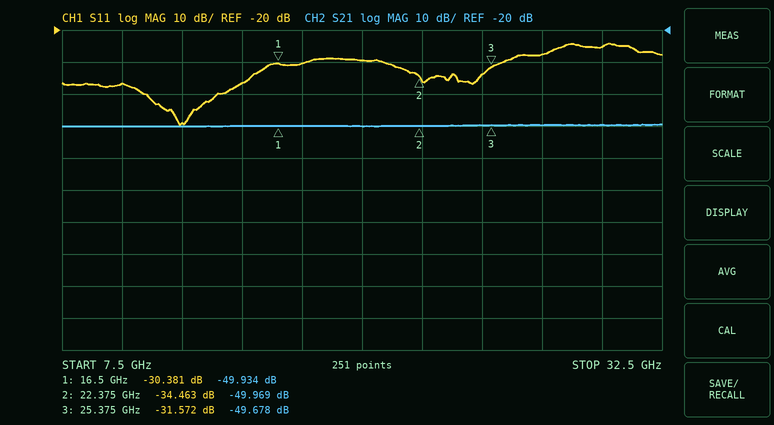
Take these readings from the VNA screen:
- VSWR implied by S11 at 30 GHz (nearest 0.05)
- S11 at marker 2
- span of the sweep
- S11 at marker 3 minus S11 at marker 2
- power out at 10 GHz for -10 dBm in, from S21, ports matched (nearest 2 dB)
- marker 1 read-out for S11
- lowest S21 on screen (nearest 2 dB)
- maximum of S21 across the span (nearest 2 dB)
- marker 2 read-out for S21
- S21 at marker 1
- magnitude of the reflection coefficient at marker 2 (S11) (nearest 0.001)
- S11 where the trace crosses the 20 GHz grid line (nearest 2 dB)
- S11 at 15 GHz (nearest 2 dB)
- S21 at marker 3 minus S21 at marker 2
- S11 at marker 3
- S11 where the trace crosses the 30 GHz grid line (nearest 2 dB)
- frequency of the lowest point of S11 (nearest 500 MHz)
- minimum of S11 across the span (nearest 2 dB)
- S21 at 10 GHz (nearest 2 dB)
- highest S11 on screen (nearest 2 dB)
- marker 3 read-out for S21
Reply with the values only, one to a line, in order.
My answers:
1.10
-34.463 dB
25 GHz
2.891 dB
-60 dBm
-30.381 dB
-50 dB
-50 dB
-49.969 dB
-49.934 dB
0.019
-30 dB
-36 dB
0.291 dB
-31.572 dB
-26 dB
12.5 GHz
-50 dB
-50 dB
-24 dB
-49.678 dB
